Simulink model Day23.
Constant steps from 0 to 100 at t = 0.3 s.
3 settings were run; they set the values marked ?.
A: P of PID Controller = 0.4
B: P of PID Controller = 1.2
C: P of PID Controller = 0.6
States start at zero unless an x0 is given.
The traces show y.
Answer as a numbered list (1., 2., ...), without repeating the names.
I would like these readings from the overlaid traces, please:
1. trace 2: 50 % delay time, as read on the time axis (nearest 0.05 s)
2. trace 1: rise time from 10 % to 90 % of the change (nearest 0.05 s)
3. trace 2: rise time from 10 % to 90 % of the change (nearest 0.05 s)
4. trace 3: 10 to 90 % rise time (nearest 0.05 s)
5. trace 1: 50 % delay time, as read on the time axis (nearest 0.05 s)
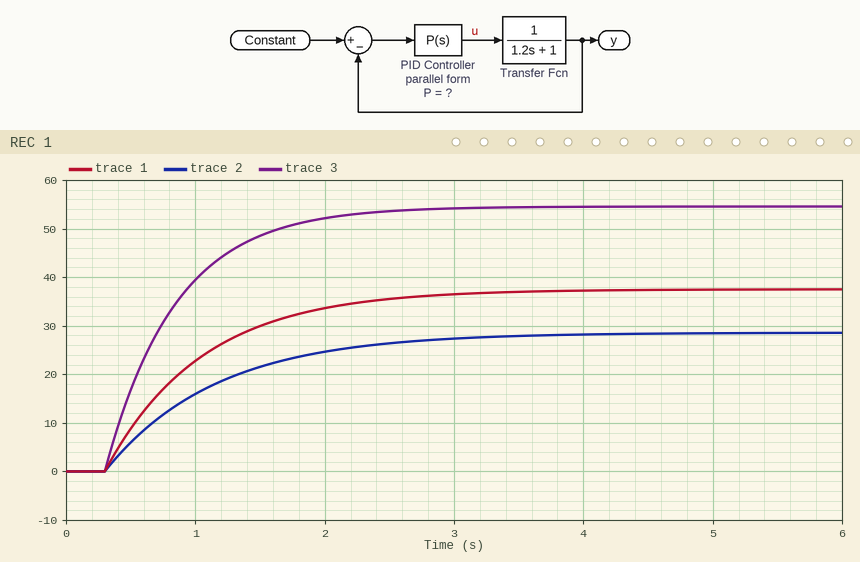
1. 0.90 s
2. 1.65 s
3. 1.90 s
4. 1.20 s
5. 0.80 s
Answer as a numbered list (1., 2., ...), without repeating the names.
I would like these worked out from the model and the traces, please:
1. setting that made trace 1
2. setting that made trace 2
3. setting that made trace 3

1. C
2. A
3. B
